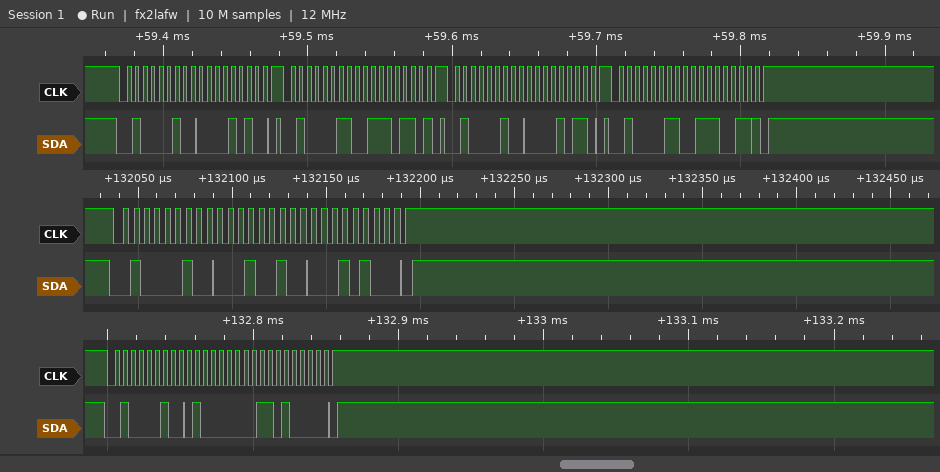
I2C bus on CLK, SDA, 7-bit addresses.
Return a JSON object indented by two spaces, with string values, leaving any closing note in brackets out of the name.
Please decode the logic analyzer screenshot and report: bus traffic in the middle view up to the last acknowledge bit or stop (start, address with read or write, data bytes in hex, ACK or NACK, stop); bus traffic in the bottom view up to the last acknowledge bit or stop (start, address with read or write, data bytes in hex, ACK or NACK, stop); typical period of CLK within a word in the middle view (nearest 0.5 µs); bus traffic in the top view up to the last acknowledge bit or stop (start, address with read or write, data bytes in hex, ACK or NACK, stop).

{
  "bus traffic in the middle view up to the last acknowledge bit or stop": "start, address 21 write ACK, 12 ACK, 14 ACK, stop",
  "bus traffic in the bottom view up to the last acknowledge bit or stop": "start, address 21 write ACK, 40 ACK, D0 ACK, stop",
  "typical period of CLK within a word in the middle view": "5.5 µs",
  "bus traffic in the top view up to the last acknowledge bit or stop": "start, address 21 write ACK, 0A ACK, stop, start, address 21 read ACK, 76 NACK, stop, start, address 21 write ACK, 0B ACK, stop, start, address 21 read ACK, 73 NACK, stop"
}
